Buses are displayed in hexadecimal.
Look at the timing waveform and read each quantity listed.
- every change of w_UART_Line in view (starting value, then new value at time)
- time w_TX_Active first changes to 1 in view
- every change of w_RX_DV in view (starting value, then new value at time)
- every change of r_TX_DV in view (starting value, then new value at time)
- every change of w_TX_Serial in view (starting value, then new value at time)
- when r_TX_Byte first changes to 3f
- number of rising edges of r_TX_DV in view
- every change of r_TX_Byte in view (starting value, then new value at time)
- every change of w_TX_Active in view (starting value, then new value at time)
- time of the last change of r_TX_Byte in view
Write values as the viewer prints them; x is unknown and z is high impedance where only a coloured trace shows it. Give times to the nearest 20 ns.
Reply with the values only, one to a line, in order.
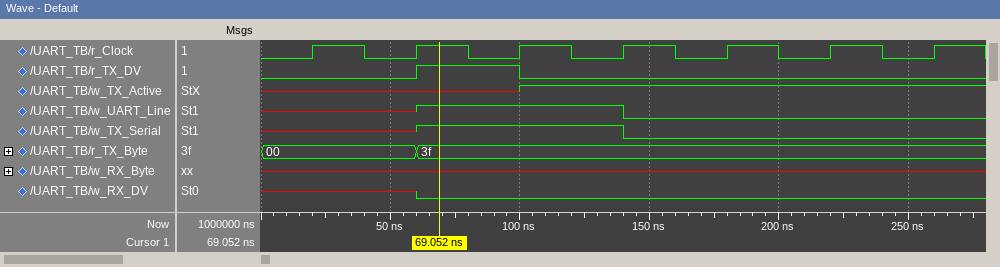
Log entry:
x, 1 at 60 ns, 0 at 140 ns
100 ns
x, 0 at 60 ns
0, 1 at 60 ns, 0 at 100 ns
x, 1 at 60 ns, 0 at 140 ns
60 ns
1
00, 3f at 60 ns
x, 1 at 100 ns
60 ns
